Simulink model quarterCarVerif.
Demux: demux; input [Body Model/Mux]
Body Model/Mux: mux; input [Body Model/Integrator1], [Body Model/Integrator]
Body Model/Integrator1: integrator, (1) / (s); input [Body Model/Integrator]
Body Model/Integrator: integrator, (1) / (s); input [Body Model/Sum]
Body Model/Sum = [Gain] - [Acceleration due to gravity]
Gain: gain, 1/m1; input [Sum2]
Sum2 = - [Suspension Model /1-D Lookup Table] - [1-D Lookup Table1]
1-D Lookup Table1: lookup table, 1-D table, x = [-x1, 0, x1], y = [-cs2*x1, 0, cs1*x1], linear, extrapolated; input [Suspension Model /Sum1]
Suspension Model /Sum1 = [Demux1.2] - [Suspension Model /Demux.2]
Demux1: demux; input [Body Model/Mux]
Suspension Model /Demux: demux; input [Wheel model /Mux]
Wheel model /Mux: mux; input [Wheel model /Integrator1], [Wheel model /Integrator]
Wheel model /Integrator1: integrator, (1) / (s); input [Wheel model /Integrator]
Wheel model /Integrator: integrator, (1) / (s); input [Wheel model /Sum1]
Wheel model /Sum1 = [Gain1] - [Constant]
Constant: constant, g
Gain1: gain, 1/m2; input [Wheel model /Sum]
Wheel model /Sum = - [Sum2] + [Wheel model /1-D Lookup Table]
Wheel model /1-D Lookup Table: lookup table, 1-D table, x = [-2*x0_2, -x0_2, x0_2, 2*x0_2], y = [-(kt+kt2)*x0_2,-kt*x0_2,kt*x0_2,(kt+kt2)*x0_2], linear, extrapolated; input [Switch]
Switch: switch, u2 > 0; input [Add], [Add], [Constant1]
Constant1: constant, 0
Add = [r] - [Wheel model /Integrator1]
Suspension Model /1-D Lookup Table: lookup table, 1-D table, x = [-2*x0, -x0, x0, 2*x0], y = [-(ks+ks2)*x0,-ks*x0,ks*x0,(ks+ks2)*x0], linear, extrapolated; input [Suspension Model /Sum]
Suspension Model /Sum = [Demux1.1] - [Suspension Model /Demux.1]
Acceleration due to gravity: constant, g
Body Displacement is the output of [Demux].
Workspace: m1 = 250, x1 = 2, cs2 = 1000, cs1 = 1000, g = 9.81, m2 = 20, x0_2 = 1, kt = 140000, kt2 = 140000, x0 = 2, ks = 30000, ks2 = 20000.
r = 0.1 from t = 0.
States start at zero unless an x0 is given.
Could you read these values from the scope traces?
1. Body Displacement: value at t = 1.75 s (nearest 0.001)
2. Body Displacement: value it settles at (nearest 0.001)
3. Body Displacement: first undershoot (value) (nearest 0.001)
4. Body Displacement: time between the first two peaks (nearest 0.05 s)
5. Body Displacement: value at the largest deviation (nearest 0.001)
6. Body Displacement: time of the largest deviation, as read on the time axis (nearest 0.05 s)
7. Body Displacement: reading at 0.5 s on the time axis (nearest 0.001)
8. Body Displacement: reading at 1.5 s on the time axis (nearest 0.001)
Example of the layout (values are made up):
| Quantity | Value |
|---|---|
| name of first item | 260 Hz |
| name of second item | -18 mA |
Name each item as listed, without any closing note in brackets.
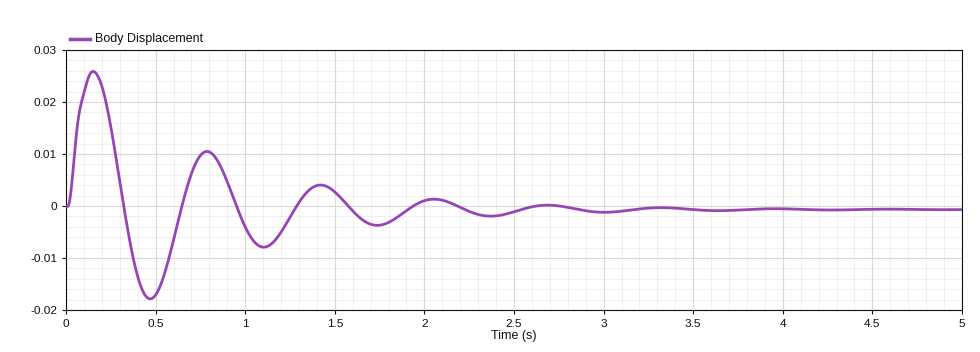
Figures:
| Quantity | Value |
|---|---|
| Body Displacement: value at t = 1.75 s | -0.004 |
| Body Displacement: value it settles at | -0.001 |
| Body Displacement: first undershoot (value) | -0.018 |
| Body Displacement: time between the first two peaks | 0.65 s |
| Body Displacement: value at the largest deviation | 0.026 |
| Body Displacement: time of the largest deviation, as read on the time axis | 0.15 s |
| Body Displacement: reading at 0.5 s on the time axis | -0.017 |
| Body Displacement: reading at 1.5 s on the time axis | 0.003 |
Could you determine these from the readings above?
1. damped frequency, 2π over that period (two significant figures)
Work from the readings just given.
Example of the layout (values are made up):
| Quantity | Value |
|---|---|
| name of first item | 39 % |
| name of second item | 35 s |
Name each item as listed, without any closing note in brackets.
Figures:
| Quantity | Value |
|---|---|
| damped frequency, 2π over that period | 9.7 rad/s |
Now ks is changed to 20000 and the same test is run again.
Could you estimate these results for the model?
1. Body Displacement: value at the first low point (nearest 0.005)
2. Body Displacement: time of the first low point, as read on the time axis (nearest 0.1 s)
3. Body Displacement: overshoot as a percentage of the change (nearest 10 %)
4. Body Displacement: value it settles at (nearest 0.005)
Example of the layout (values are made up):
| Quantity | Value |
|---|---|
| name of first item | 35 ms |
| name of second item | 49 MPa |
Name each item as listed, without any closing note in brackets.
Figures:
| Quantity | Value |
|---|---|
| Body Displacement: value at the first low point | -0.075 |
| Body Displacement: time of the first low point, as read on the time axis | 0.5 s |
| Body Displacement: overshoot as a percentage of the change | 80 % |
| Body Displacement: value it settles at | -0.040 |
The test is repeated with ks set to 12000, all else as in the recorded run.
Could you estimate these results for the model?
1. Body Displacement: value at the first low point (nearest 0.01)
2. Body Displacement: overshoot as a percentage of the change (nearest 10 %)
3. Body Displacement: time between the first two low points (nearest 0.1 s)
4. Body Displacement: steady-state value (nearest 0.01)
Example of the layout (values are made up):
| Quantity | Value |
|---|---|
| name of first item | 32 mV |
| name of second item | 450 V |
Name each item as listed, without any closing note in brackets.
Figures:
| Quantity | Value |
|---|---|
| Body Displacement: value at the first low point | -0.18 |
| Body Displacement: overshoot as a percentage of the change | 50 % |
| Body Displacement: time between the first two low points | 1.0 s |
| Body Displacement: steady-state value | -0.12 |
